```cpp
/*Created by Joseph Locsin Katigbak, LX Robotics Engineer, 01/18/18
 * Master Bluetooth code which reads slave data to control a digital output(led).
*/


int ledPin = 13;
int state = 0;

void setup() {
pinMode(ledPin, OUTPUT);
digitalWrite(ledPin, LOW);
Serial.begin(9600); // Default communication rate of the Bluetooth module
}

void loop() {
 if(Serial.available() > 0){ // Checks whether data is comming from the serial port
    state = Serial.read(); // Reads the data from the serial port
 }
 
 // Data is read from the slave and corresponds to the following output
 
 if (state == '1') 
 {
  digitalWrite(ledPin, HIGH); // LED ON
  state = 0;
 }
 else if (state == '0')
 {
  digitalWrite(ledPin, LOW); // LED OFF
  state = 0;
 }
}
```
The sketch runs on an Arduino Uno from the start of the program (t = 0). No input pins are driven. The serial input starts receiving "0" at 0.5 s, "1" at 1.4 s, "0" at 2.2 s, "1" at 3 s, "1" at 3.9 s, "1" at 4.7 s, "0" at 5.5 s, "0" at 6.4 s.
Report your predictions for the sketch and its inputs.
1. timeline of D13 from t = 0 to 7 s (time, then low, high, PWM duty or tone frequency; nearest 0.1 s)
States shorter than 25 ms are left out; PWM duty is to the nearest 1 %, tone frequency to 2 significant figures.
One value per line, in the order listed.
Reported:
0 s low; 1.4 s high; 2.2 s low; 3 s high; 5.5 s low
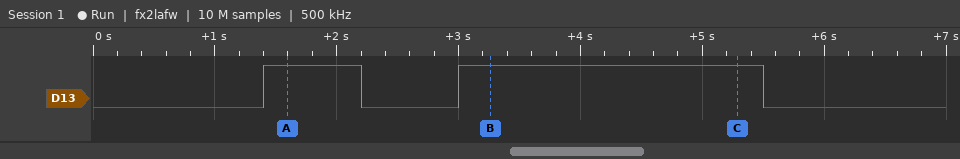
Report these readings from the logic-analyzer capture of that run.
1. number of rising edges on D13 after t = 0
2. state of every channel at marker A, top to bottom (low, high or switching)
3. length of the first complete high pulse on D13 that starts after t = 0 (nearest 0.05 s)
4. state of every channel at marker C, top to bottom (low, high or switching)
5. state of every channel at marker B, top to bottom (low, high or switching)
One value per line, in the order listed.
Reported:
2
D13 high
0.80 s
D13 high
D13 high
